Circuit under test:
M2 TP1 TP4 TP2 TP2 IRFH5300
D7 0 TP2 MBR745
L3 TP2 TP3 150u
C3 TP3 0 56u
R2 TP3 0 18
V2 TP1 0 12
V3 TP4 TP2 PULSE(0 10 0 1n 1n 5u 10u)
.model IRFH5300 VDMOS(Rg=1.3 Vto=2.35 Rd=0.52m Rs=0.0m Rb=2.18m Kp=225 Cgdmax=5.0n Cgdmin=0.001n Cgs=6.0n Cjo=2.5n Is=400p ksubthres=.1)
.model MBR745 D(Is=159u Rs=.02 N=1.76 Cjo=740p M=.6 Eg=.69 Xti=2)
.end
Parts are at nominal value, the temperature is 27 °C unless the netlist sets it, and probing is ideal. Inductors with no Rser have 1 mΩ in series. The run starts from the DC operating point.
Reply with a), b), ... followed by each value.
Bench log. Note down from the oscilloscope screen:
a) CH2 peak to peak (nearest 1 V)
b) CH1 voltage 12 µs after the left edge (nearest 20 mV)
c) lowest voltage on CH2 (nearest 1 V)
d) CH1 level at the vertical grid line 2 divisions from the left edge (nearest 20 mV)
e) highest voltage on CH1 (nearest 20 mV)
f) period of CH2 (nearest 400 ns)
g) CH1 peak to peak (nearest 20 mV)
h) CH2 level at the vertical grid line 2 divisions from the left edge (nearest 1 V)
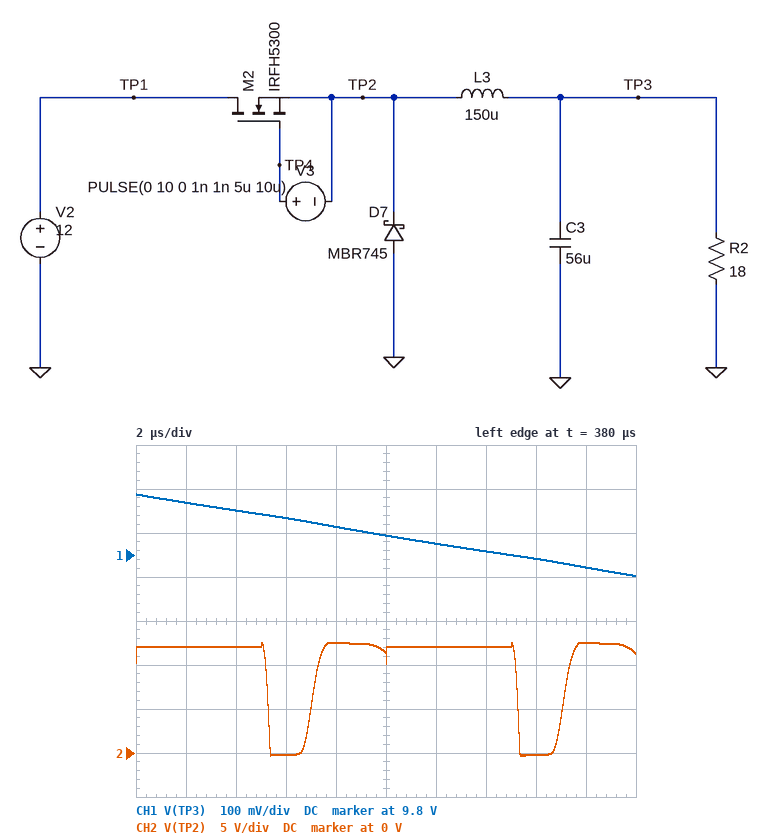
a) 13 V
b) 9.82 V
c) 0 V
d) 9.90 V
e) 9.94 V
f) 10.0 µs
g) 180 mV
h) 12 V
